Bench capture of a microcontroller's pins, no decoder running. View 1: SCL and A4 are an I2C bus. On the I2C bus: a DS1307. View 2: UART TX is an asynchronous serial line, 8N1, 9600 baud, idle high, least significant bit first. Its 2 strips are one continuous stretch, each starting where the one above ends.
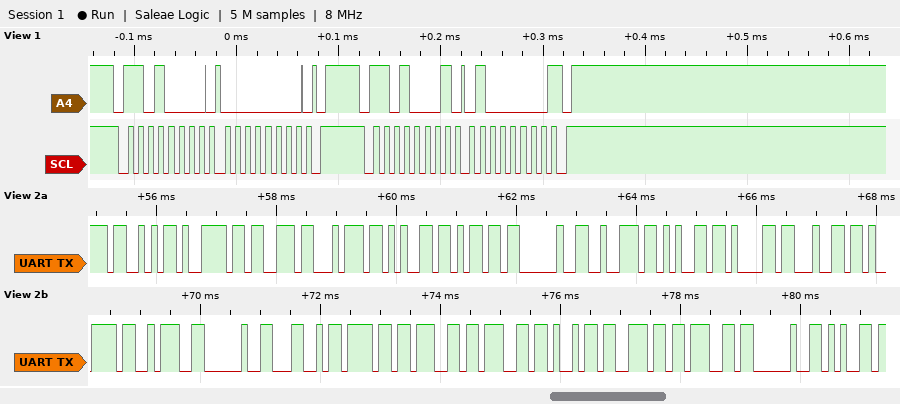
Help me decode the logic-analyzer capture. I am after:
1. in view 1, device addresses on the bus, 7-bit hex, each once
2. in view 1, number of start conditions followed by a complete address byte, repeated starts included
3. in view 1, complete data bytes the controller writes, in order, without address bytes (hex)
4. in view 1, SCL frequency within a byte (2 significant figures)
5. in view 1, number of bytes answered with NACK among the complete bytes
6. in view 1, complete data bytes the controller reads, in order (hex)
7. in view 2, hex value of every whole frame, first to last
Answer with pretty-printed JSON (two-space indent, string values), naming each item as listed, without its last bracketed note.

{
  "in view 1, device addresses on the bus, 7-bit hex, each once": "0x68",
  "in view 1, number of start conditions followed by a complete address byte, repeated starts included": "2",
  "in view 1, complete data bytes the controller writes, in order, without address bytes": "00",
  "in view 1, SCL frequency within a byte": "100 kHz",
  "in view 1, number of bytes answered with NACK among the complete bytes": "1",
  "in view 1, complete data bytes the controller reads, in order": "40",
  "in view 2, hex value of every whole frame, first to last": "0x53 0x79 0x73 0x74 0x65 0x6D 0x20 0x72 0x65 0x61 0x64 0x79 0x3A 0x20 0x4C 0x6F 0x67 0x67 0x69 0x6E 0x67 0x20 0x65"
}
